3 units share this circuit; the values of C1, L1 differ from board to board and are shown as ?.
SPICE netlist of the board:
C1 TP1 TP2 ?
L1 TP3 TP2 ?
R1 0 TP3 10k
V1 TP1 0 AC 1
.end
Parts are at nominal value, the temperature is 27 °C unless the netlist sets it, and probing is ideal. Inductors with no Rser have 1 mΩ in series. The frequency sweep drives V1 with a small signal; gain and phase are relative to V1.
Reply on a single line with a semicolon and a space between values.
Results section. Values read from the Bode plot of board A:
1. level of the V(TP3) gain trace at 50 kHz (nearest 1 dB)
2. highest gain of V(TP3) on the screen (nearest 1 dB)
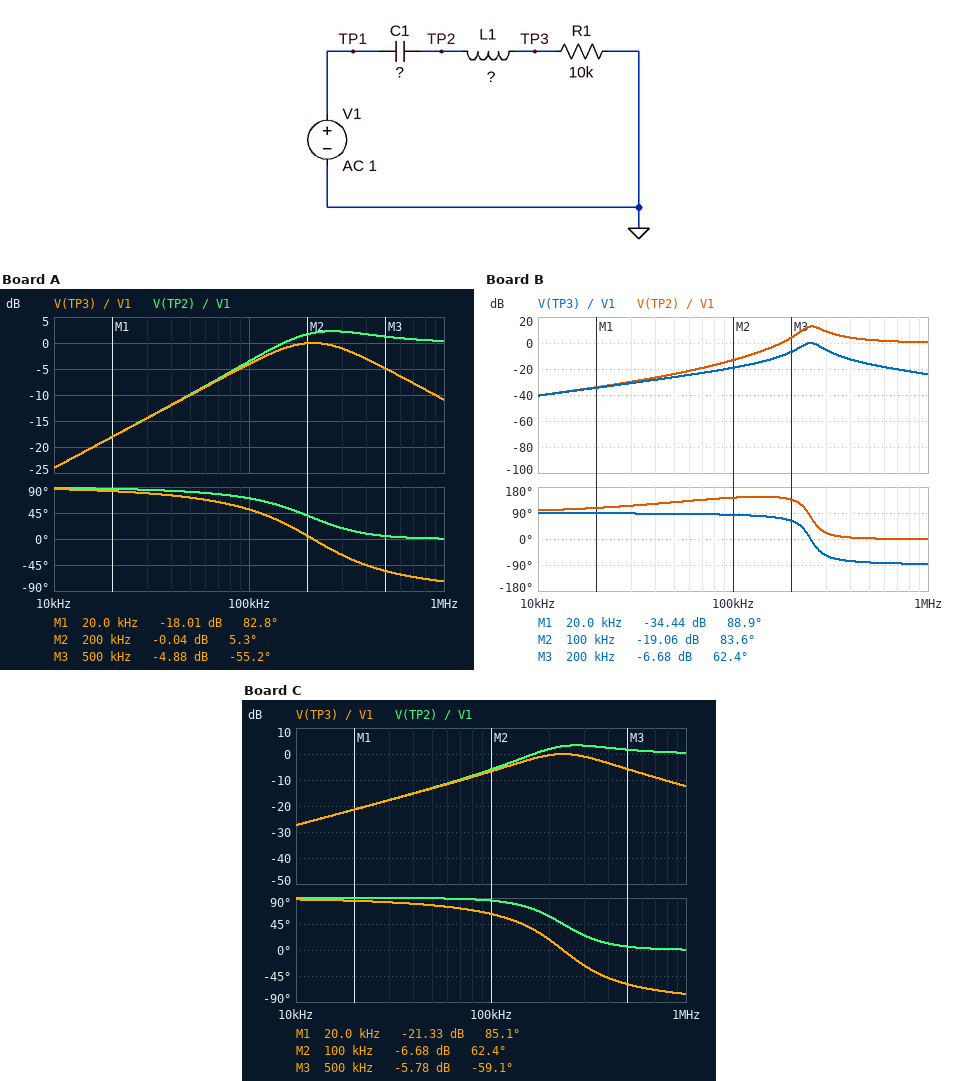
-10 dB; 0 dB
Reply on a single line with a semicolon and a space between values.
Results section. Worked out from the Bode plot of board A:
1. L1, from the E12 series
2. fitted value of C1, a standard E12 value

5.6 mH; 100 pF
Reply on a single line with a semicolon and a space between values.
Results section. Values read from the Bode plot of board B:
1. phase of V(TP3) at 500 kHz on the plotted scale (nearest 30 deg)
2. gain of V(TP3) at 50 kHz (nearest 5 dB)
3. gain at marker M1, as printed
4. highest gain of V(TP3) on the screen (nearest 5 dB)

-90 deg; -25 dB; -34.44 dB; 0 dB
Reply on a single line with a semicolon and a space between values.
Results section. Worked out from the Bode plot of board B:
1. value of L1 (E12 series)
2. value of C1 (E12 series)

27 mH; 15 pF
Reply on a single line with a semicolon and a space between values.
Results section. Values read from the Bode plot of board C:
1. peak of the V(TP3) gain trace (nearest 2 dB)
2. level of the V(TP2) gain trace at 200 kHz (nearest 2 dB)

0 dB; 2 dB
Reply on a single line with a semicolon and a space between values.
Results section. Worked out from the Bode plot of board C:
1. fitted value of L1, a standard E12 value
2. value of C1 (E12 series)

6.8 mH; 68 pF
